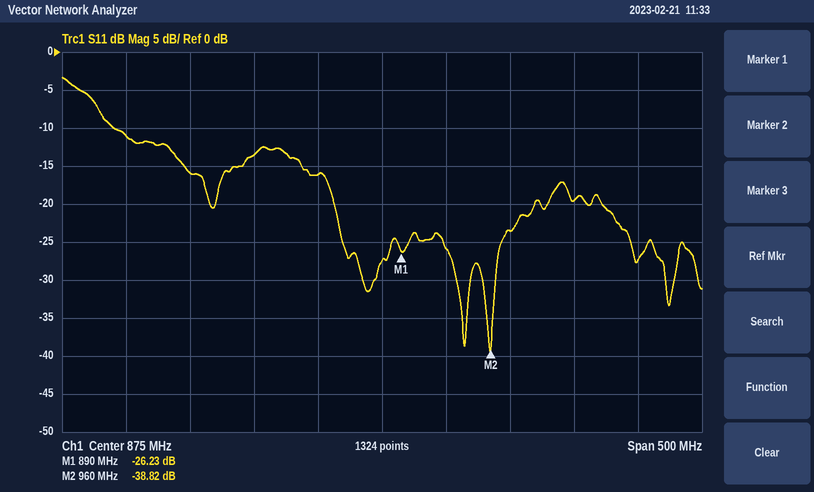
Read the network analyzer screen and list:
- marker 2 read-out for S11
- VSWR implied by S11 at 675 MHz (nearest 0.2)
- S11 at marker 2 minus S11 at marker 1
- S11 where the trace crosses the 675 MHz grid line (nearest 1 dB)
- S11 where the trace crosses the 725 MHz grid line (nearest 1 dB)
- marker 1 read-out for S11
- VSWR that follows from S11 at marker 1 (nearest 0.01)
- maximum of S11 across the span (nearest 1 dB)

-38.82 dB
1.8
-12.59 dB
-11 dB
-16 dB
-26.23 dB
1.10
-3 dB
